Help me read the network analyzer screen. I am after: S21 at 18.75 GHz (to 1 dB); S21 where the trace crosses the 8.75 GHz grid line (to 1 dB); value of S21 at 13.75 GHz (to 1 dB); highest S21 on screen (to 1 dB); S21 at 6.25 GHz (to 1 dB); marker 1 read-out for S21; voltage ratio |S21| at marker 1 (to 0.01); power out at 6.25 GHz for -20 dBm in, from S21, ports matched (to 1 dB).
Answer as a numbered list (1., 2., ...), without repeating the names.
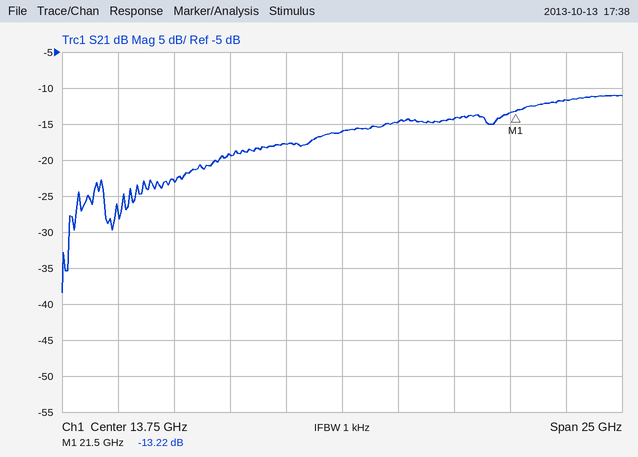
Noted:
1. -14 dB
2. -19 dB
3. -16 dB
4. -11 dB
5. -23 dB
6. -13.22 dB
7. 0.22
8. -43 dBm
